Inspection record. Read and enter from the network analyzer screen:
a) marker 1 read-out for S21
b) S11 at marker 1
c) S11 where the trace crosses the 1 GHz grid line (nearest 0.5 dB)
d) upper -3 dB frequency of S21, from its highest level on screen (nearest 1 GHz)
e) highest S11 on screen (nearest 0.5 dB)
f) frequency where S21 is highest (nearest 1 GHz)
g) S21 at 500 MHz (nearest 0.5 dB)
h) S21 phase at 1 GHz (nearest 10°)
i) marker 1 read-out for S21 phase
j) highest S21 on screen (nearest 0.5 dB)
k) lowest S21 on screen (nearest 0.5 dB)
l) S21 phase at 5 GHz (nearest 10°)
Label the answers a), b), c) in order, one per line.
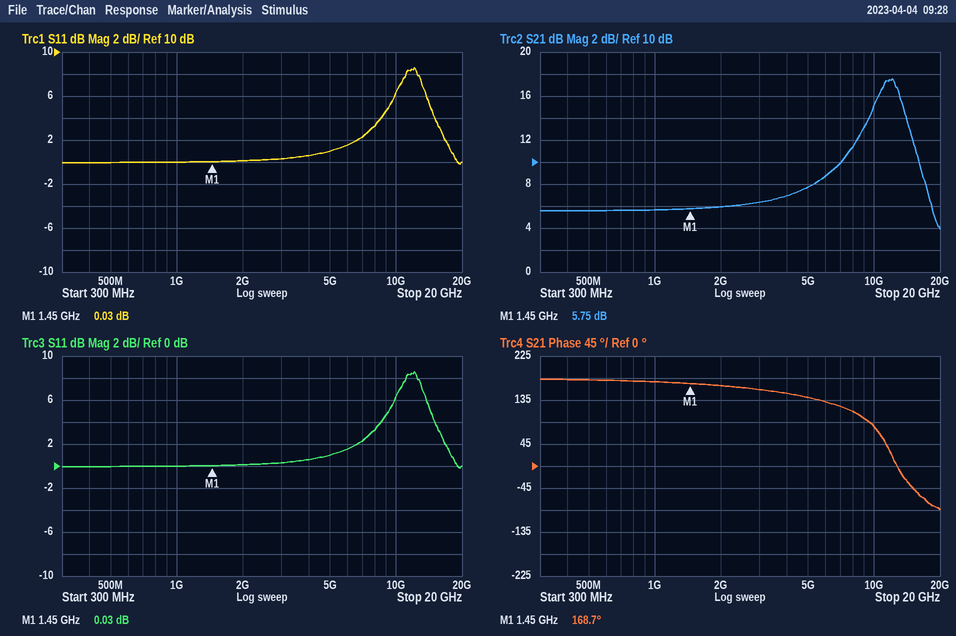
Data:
a) 5.75 dB
b) 0.03 dB
c) 0.0 dB
d) 14 GHz
e) 8.5 dB
f) 12 GHz
g) 5.5 dB
h) 170°
i) 168.7°
j) 17.5 dB
k) 4.0 dB
l) 140°
